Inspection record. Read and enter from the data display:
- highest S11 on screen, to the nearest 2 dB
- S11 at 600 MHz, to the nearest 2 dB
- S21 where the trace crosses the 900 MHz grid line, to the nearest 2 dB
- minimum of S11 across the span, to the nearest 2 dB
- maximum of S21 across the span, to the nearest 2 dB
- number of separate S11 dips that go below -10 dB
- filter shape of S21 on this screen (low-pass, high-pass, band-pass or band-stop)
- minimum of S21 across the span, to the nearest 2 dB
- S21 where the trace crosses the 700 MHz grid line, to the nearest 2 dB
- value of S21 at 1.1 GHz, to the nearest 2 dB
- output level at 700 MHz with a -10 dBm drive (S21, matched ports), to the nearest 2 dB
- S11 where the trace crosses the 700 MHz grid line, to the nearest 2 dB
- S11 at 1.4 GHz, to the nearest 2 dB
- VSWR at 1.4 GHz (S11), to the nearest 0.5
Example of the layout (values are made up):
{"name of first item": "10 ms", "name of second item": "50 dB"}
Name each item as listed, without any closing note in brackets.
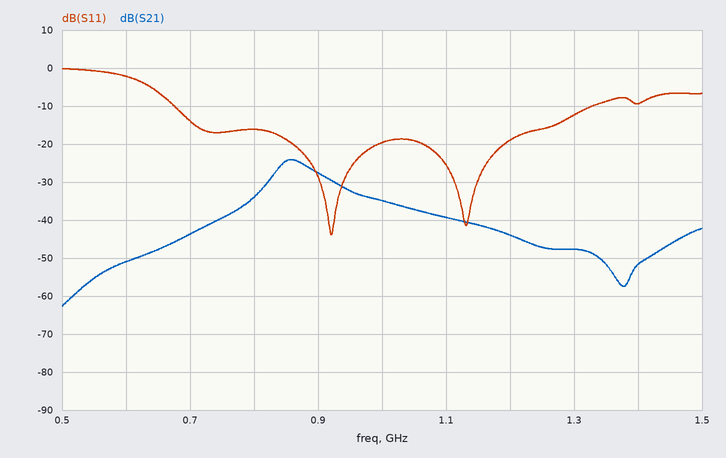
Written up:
{"highest S11 on screen, to the nearest 2 dB": "0 dB", "S11 at 600 MHz, to the nearest 2 dB": "-2 dB", "S21 where the trace crosses the 900 MHz grid line, to the nearest 2 dB": "-28 dB", "minimum of S11 across the span, to the nearest 2 dB": "-44 dB", "maximum of S21 across the span, to the nearest 2 dB": "-24 dB", "number of separate S11 dips that go below -10 dB": "2", "filter shape of S21 on this screen": "band-pass", "minimum of S21 across the span, to the nearest 2 dB": "-62 dB", "S21 where the trace crosses the 700 MHz grid line, to the nearest 2 dB": "-44 dB", "value of S21 at 1.1 GHz, to the nearest 2 dB": "-40 dB", "output level at 700 MHz with a -10 dBm drive (S21, matched ports), to the nearest 2 dB": "-54 dBm", "S11 where the trace crosses the 700 MHz grid line, to the nearest 2 dB": "-14 dB", "S11 at 1.4 GHz, to the nearest 2 dB": "-10 dB", "VSWR at 1.4 GHz (S11), to the nearest 0.5": "2.0"}
